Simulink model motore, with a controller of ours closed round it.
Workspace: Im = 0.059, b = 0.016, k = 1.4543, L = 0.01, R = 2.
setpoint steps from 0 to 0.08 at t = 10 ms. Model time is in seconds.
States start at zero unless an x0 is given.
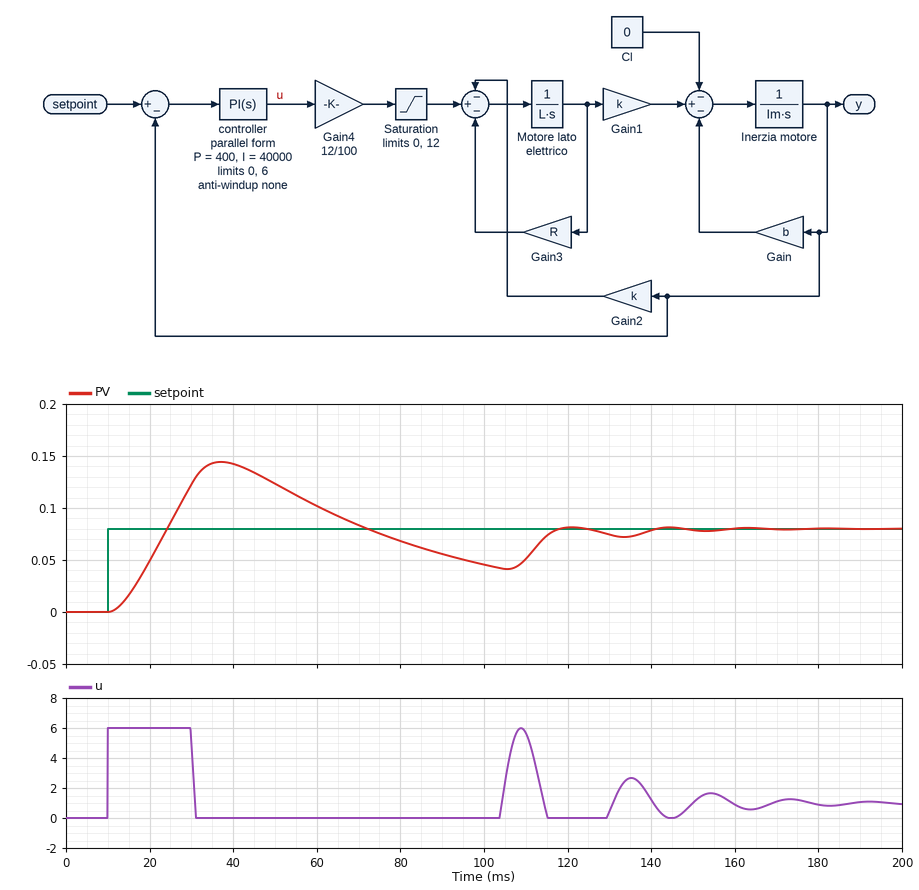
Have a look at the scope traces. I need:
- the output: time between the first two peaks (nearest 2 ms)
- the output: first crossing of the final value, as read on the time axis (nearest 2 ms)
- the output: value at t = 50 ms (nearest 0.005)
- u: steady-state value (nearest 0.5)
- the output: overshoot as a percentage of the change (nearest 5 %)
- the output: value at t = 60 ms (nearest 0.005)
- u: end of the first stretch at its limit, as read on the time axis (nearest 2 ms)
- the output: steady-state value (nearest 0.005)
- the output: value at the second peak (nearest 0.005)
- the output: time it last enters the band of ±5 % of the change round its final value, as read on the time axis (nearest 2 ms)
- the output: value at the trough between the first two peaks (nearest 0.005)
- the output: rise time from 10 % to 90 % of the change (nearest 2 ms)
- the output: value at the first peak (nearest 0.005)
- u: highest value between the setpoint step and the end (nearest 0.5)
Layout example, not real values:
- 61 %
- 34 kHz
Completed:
- 84 ms
- 24 ms
- 0.125
- 1.0
- 80 %
- 0.100
- 30 ms
- 0.080
- 0.080
- 138 ms
- 0.040
- 10 ms
- 0.145
- 6.0
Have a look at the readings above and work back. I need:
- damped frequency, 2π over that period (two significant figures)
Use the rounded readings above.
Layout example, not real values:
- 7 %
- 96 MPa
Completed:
- 0.075 rad/ms
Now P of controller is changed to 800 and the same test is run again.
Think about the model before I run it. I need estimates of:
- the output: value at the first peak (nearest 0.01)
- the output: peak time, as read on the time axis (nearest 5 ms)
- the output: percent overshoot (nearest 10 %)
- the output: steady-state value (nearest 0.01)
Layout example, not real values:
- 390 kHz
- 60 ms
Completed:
- 0.13
- 35 ms
- 60 %
- 0.08
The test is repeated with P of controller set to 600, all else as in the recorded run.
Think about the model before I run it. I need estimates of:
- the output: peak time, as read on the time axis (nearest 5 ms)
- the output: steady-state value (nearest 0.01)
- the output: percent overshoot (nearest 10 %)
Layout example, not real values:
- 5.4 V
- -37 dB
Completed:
- 35 ms
- 0.08
- 70 %
